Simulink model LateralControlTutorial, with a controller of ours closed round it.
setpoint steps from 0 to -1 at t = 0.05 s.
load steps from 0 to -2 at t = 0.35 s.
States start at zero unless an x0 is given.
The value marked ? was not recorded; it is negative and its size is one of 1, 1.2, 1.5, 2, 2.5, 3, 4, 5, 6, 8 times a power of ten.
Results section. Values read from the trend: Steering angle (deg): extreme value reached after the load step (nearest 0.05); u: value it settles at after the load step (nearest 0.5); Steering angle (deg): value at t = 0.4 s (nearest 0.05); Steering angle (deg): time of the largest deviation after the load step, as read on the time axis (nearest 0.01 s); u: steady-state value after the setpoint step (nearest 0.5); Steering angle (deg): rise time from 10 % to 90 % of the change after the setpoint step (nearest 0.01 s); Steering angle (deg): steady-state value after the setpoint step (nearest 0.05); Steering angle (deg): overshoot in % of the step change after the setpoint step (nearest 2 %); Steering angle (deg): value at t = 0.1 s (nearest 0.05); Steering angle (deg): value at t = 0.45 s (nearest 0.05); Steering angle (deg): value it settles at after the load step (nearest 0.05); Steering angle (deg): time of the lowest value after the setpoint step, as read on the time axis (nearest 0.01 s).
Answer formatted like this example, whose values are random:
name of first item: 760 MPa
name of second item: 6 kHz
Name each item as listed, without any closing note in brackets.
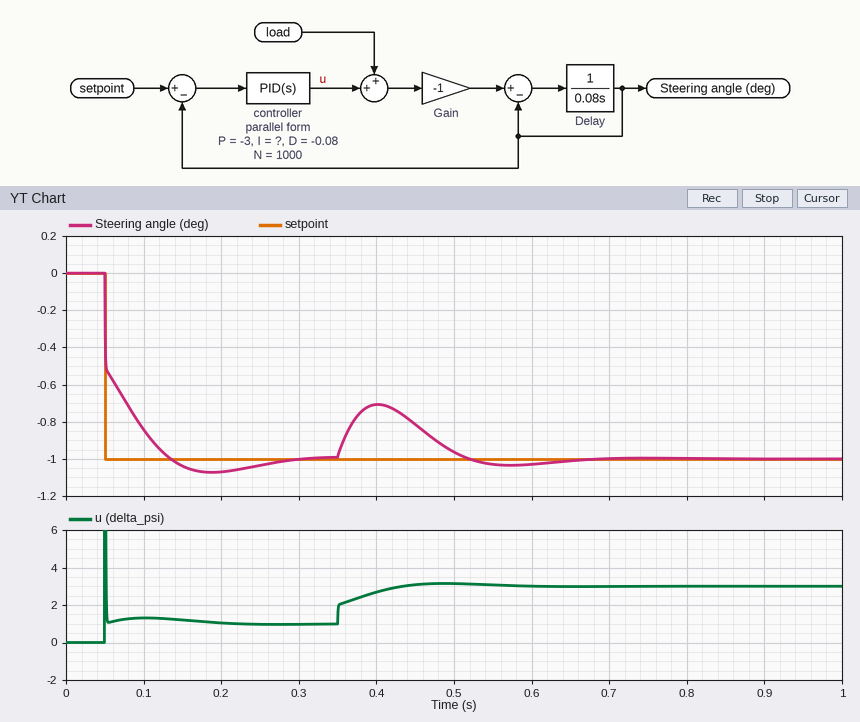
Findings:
Steering angle (deg): extreme value reached after the load step: -0.70
u: value it settles at after the load step: 3.0
Steering angle (deg): value at t = 0.4 s: -0.70
Steering angle (deg): time of the largest deviation after the load step, as read on the time axis: 0.40 s
u: steady-state value after the setpoint step: 1.0
Steering angle (deg): rise time from 10 % to 90 % of the change after the setpoint step: 0.06 s
Steering angle (deg): steady-state value after the setpoint step: -1.00
Steering angle (deg): overshoot in % of the step change after the setpoint step: 8 %
Steering angle (deg): value at t = 0.1 s: -0.85
Steering angle (deg): value at t = 0.45 s: -0.80
Steering angle (deg): value it settles at after the load step: -1.00
Steering angle (deg): time of the lowest value after the setpoint step, as read on the time axis: 0.19 s
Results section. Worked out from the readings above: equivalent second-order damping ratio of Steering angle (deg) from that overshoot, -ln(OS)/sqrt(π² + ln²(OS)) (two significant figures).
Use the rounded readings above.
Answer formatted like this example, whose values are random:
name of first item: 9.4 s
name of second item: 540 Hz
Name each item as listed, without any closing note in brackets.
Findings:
equivalent second-order damping ratio of Steering angle (deg) from that overshoot, -ln(OS)/sqrt(π² + ln²(OS)): 0.63
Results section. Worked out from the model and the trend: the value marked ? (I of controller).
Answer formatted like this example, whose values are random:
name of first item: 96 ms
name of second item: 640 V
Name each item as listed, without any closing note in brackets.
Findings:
the value marked ?: -80
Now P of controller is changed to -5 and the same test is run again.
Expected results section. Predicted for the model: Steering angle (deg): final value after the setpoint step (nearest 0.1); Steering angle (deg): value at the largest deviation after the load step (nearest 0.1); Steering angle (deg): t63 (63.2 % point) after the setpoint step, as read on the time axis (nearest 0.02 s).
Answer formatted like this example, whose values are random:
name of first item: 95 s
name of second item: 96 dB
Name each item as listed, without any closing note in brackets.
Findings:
Steering angle (deg): final value after the setpoint step: -1.0
Steering angle (deg): value at the largest deviation after the load step: -0.8
Steering angle (deg): t63 (63.2 % point) after the setpoint step, as read on the time axis: 0.06 s
